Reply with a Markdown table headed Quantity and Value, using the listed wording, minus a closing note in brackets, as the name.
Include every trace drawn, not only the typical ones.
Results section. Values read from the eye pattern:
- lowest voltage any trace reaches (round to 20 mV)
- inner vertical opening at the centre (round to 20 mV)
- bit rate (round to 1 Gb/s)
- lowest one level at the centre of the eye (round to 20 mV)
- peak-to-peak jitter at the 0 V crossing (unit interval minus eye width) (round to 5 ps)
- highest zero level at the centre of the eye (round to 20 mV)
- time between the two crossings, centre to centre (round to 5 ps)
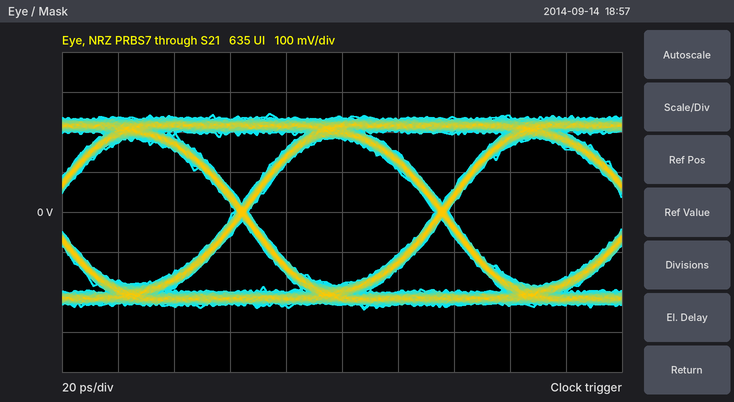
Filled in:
| Quantity | Value |
|---|---|
| lowest voltage any trace reaches | -240 mV |
| inner vertical opening at the centre | 360 mV |
| bit rate | 14 Gb/s |
| lowest one level at the centre of the eye | 180 mV |
| peak-to-peak jitter at the 0 V crossing (unit interval minus eye width) | 5 ps |
| highest zero level at the centre of the eye | -180 mV |
| time between the two crossings, centre to centre | 70 ps |
